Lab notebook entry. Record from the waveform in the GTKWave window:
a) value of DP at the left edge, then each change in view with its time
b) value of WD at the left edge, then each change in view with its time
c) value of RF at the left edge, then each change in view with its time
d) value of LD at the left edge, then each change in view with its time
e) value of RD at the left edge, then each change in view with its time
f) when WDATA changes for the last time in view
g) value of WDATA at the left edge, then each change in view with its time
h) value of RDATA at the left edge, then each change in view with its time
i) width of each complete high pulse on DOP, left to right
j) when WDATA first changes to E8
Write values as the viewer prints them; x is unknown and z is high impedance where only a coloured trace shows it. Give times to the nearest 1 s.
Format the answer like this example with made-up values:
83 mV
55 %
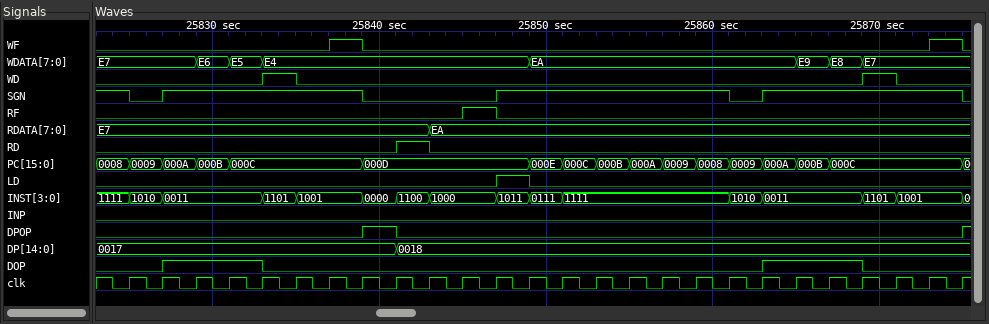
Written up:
0017, 0018 at 25841 s
0, 1 at 25833 s, 0 at 25835 s, 1 at 25869 s, 0 at 25871 s
0, 1 at 25845 s, 0 at 25847 s
0, 1 at 25847 s, 0 at 25849 s
0, 1 at 25841 s, 0 at 25843 s
25869 s
E7, E6 at 25829 s, E5 at 25831 s, E4 at 25833 s, EA at 25849 s, E9 at 25865 s, E8 at 25867 s, E7 at 25869 s
E7, EA at 25843 s
6 s, 6 s
25867 s
